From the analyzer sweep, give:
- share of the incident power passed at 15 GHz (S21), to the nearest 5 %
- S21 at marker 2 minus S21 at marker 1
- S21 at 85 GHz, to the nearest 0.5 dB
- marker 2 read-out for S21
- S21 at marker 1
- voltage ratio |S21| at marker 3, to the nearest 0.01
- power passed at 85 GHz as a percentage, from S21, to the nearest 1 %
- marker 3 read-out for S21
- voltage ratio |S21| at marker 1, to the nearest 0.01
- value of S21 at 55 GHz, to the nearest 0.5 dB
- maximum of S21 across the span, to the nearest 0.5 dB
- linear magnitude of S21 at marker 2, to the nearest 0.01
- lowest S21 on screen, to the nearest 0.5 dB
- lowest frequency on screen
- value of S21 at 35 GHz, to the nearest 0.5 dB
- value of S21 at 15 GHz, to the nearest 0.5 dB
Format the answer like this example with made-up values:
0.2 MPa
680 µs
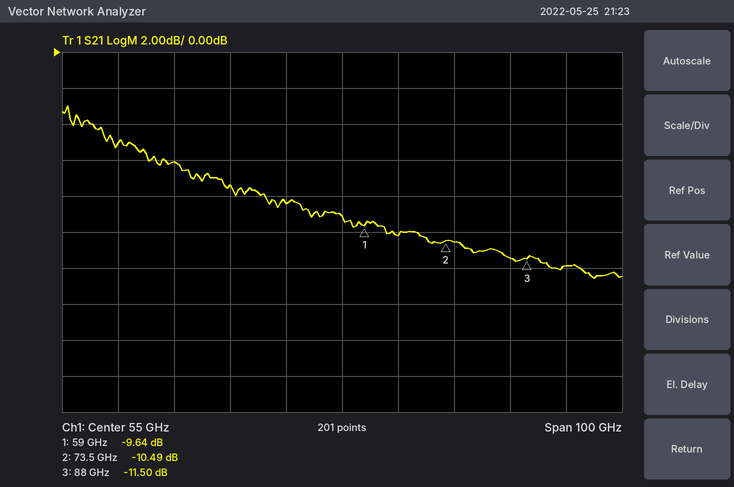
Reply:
30 %
-0.85 dB
-11.5 dB
-10.49 dB
-9.64 dB
0.27
7 %
-11.50 dB
0.33
-9.0 dB
-3.0 dB
0.30
-12.5 dB
5 GHz
-7.5 dB
-5.0 dB
